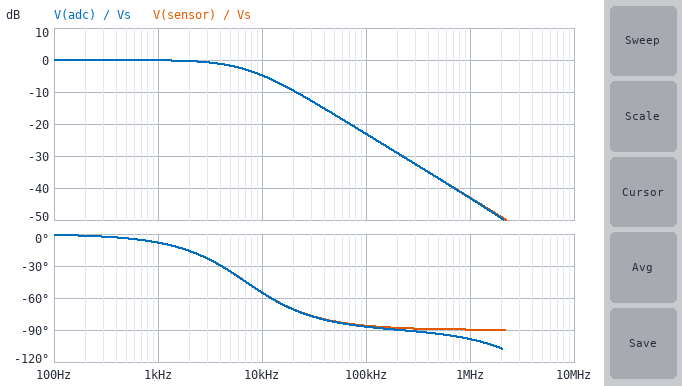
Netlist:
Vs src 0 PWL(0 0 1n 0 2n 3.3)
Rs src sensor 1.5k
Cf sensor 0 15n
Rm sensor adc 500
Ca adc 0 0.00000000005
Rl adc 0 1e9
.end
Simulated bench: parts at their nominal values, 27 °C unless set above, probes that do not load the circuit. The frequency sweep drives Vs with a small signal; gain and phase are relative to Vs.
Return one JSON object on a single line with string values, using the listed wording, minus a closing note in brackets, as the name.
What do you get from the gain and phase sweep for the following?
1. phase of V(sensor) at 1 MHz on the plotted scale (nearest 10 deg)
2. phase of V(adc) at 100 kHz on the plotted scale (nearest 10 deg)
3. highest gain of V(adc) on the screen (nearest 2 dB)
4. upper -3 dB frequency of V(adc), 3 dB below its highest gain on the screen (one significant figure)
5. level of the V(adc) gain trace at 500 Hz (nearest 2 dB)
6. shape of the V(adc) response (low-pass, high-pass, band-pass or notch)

{"phase of V(sensor) at 1 MHz on the plotted scale": "-90 deg", "phase of V(adc) at 100 kHz on the plotted scale": "-90 deg", "highest gain of V(adc) on the screen": "0 dB", "upper -3 dB frequency of V(adc), 3 dB below its highest gain on the screen": "7 kHz", "level of the V(adc) gain trace at 500 Hz": "0 dB", "shape of the V(adc) response": "low-pass"}
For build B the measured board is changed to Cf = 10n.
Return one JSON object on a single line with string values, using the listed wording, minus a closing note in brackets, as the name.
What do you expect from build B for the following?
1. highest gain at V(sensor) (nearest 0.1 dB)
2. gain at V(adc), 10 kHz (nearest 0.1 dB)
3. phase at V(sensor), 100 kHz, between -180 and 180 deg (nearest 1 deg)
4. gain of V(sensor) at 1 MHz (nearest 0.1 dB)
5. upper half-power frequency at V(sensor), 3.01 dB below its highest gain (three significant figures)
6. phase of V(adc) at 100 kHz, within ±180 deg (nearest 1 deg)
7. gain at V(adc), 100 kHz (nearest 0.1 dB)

{"highest gain at V(sensor)": "0 dB", "gain at V(adc), 10 kHz": "-2.8 dB", "phase at V(sensor), 100 kHz, between -180 and 180 deg": "-84 deg", "gain of V(sensor) at 1 MHz": "-39.5 dB", "upper half-power frequency at V(sensor), 3.01 dB below its highest gain": "10.6 kHz", "phase of V(adc) at 100 kHz, within ±180 deg": "-85 deg", "gain at V(adc), 100 kHz": "-19.6 dB"}
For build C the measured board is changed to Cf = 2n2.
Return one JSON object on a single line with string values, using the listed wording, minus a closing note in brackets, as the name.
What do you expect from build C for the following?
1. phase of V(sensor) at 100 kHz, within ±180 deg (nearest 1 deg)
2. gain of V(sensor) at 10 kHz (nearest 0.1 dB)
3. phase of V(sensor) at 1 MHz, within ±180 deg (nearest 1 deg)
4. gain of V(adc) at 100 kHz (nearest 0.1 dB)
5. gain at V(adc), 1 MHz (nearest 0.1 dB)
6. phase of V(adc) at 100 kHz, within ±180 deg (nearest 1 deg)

{"phase of V(sensor) at 100 kHz, within ±180 deg": "-65 deg", "gain of V(sensor) at 10 kHz": "-0.2 dB", "phase of V(sensor) at 1 MHz, within ±180 deg": "-87 deg", "gain of V(adc) at 100 kHz": "-7.4 dB", "gain at V(adc), 1 MHz": "-26.6 dB", "phase of V(adc) at 100 kHz, within ±180 deg": "-66 deg"}
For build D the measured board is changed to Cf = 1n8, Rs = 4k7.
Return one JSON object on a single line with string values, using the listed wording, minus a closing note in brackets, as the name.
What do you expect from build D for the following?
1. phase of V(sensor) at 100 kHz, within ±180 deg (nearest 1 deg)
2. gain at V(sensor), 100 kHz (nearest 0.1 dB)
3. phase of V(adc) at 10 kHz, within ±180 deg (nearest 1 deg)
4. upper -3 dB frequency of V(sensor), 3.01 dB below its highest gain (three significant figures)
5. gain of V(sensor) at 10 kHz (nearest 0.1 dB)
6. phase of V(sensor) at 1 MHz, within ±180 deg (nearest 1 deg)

{"phase of V(sensor) at 100 kHz, within ±180 deg": "-80 deg", "gain at V(sensor), 100 kHz": "-14.9 dB", "phase of V(adc) at 10 kHz, within ±180 deg": "-29 deg", "upper -3 dB frequency of V(sensor), 3.01 dB below its highest gain": "18.3 kHz", "gain of V(sensor) at 10 kHz": "-1.1 dB", "phase of V(sensor) at 1 MHz, within ±180 deg": "-89 deg"}
